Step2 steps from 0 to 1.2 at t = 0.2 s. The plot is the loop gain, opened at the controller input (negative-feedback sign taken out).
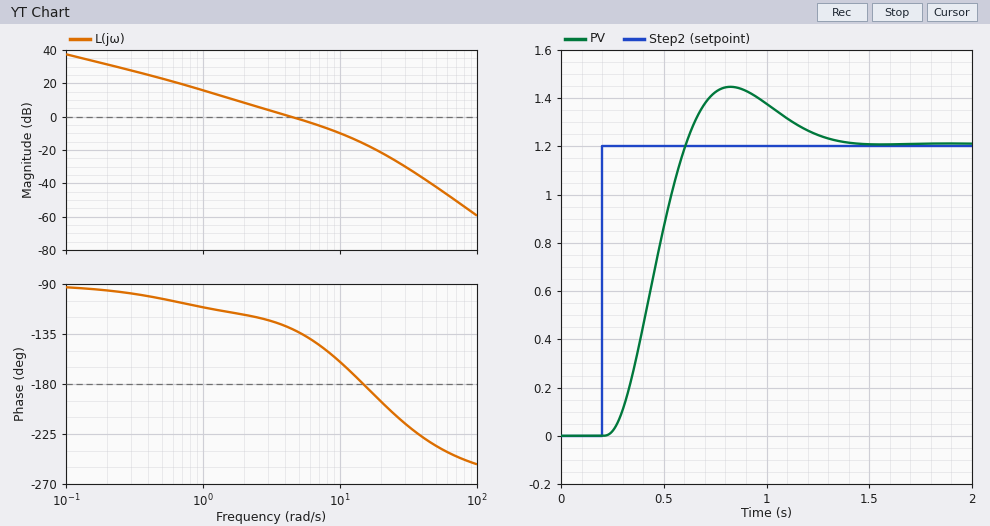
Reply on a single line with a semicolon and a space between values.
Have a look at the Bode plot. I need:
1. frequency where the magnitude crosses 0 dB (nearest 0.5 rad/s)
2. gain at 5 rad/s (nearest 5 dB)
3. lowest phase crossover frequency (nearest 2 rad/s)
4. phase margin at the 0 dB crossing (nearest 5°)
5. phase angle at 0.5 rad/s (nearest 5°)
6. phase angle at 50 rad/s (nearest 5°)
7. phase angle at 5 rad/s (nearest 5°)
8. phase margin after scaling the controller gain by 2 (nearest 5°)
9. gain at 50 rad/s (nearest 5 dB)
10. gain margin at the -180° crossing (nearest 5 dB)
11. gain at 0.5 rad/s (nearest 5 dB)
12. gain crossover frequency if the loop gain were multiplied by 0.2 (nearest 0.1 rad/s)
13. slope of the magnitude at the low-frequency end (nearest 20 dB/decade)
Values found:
4.5 rad/s; 0 dB; 14 rad/s; 50°; -105°; -235°; -135°; 35°; -40 dB; 15 dB; 25 dB; 1.2 rad/s; -20 dB/decade
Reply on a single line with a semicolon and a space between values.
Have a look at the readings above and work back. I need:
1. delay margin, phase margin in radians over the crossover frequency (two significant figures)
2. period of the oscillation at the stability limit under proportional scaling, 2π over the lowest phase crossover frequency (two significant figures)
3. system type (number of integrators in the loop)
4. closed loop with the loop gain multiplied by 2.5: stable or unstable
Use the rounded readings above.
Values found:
0.19 s; 0.45 s; 1; stable
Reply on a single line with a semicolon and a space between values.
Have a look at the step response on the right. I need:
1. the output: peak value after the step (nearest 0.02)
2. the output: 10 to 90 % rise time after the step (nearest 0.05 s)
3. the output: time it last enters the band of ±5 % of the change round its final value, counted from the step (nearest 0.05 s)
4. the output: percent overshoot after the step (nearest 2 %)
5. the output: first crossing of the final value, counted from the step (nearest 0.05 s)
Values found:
1.44; 0.25 s; 1.00 s; 20 %; 0.40 s
